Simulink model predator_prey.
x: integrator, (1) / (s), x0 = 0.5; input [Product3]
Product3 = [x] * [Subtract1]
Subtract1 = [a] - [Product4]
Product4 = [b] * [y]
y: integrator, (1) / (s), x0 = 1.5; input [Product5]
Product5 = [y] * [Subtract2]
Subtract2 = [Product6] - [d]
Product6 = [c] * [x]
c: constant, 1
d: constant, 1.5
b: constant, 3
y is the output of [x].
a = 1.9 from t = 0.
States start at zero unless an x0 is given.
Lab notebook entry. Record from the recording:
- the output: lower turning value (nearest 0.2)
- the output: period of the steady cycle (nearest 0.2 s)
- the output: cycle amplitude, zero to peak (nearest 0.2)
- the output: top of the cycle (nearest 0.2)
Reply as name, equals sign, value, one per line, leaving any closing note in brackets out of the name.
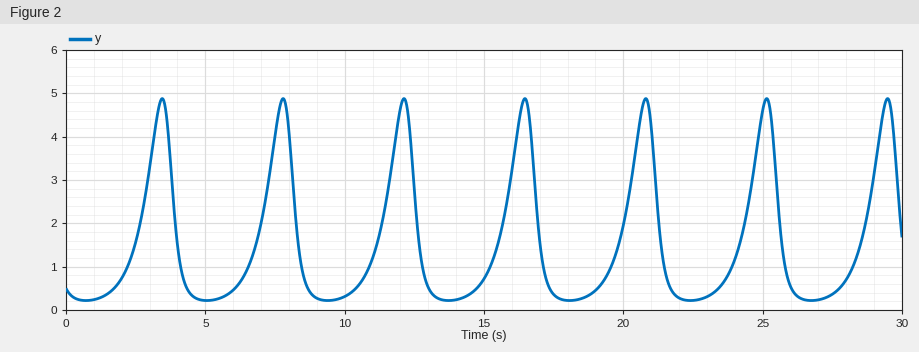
the output: lower turning value = 0.2
the output: period of the steady cycle = 4.4 s
the output: cycle amplitude, zero to peak = 2.4
the output: top of the cycle = 4.8
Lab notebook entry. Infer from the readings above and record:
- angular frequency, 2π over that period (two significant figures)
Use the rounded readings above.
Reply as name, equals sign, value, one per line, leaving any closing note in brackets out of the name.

angular frequency, 2π over that period = 1.4 rad/s
